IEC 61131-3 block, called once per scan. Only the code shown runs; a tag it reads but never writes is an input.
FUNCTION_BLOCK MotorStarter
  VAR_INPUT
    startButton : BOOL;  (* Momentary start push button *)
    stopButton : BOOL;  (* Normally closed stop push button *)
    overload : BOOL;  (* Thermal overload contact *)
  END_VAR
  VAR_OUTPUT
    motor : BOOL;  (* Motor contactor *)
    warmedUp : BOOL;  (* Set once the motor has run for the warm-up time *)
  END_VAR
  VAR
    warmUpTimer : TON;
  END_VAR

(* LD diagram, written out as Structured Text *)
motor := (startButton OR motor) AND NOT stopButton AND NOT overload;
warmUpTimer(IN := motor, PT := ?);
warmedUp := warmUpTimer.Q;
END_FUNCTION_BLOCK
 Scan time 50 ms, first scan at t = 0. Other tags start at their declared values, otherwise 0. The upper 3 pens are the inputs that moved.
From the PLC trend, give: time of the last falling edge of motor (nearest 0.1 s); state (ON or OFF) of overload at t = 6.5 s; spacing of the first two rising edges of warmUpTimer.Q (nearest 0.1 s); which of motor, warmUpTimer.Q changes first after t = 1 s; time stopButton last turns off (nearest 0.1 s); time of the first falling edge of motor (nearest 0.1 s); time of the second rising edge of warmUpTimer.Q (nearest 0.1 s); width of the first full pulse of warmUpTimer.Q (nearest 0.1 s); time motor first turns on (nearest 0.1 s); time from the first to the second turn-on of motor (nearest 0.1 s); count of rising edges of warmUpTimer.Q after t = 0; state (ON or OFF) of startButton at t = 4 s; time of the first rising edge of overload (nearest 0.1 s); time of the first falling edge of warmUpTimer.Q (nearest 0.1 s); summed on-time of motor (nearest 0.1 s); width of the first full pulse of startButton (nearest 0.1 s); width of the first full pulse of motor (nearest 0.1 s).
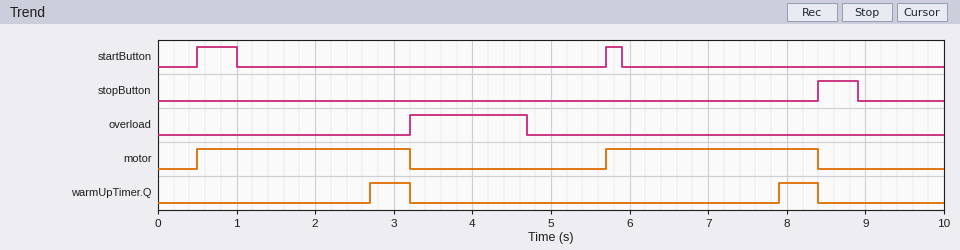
8.4 s
OFF
5.2 s
warmUpTimer.Q
8.9 s
3.2 s
7.9 s
0.5 s
0.5 s
5.2 s
2
OFF
3.2 s
3.2 s
5.4 s
0.5 s
2.7 s
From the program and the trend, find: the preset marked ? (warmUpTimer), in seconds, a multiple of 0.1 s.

2.2 s
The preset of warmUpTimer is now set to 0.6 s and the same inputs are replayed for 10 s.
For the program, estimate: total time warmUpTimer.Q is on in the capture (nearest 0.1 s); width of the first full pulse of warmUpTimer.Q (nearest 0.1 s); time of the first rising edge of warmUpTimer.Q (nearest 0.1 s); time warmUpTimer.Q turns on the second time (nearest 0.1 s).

4.2 s
2.1 s
1.1 s
6.3 s
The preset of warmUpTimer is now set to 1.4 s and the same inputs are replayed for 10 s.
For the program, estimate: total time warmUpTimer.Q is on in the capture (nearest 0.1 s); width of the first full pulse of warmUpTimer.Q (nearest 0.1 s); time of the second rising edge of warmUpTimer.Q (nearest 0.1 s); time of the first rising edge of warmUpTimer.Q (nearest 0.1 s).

2.6 s
1.3 s
7.1 s
1.9 s
